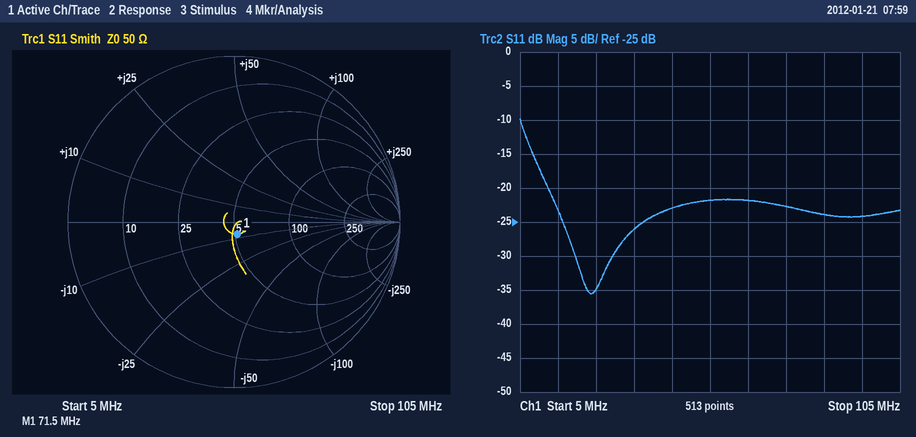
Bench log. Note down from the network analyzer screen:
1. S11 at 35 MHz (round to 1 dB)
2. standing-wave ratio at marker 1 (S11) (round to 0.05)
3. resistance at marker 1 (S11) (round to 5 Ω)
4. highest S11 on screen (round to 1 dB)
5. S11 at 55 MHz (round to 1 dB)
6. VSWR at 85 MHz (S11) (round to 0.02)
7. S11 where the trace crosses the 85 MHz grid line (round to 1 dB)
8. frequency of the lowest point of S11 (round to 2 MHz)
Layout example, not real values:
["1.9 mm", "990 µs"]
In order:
["-26 dB", "1.15", "50 Ω", "-10 dB", "-22 dB", "1.14", "-24 dB", "24 MHz"]
